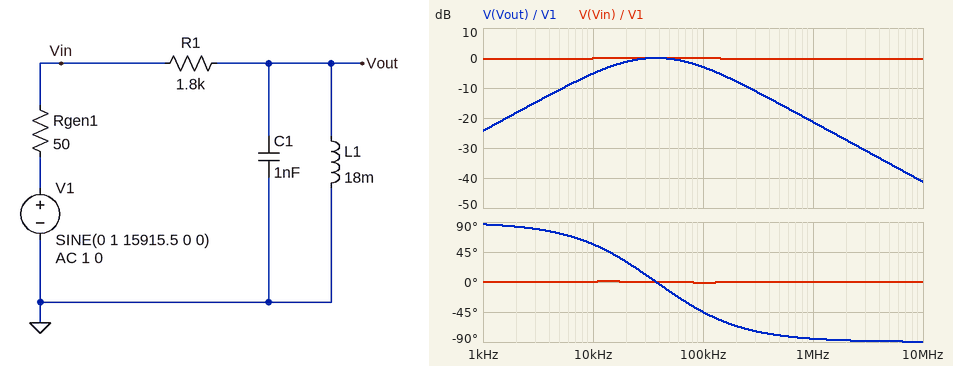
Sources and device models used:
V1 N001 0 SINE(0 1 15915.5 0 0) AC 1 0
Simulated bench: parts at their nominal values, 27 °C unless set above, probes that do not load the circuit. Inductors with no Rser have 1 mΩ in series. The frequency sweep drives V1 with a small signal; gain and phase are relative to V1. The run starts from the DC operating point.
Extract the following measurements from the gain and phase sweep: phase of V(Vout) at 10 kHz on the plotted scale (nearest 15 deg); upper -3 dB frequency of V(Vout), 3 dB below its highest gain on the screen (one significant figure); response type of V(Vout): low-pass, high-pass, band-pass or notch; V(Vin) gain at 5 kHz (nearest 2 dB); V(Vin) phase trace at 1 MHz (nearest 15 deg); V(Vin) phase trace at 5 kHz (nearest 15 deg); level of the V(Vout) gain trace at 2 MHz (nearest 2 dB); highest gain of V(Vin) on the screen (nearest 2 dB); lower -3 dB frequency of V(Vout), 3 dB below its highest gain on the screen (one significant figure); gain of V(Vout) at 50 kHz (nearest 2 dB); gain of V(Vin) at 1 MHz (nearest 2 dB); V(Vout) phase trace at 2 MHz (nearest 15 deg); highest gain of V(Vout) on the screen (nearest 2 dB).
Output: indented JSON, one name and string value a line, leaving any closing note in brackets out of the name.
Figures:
{
  "phase of V(Vout) at 10 kHz on the plotted scale": "60 deg",
  "upper -3 dB frequency of V(Vout), 3 dB below its highest gain on the screen": "100 kHz",
  "response type of V(Vout): low-pass, high-pass, band-pass or notch": "band-pass",
  "V(Vin) gain at 5 kHz": "0 dB",
  "V(Vin) phase trace at 1 MHz": "0 deg",
  "V(Vin) phase trace at 5 kHz": "0 deg",
  "level of the V(Vout) gain trace at 2 MHz": "-28 dB",
  "highest gain of V(Vin) on the screen": "0 dB",
  "lower -3 dB frequency of V(Vout), 3 dB below its highest gain on the screen": "10 kHz",
  "gain of V(Vout) at 50 kHz": "0 dB",
  "gain of V(Vin) at 1 MHz": "0 dB",
  "V(Vout) phase trace at 2 MHz": "-90 deg",
  "highest gain of V(Vout) on the screen": "0 dB"
}
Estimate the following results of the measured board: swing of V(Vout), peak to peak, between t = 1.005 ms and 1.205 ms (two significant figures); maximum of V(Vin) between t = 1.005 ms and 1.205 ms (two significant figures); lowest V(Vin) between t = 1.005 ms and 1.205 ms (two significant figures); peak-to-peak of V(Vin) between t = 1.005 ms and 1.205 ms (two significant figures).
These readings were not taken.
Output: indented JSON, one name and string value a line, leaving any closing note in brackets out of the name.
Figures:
{
  "swing of V(Vout), peak to peak, between t = 1.005 ms and 1.205 ms": "1.5 V",
  "maximum of V(Vin) between t = 1.005 ms and 1.205 ms": "990 mV",
  "lowest V(Vin) between t = 1.005 ms and 1.205 ms": "-990 mV",
  "peak-to-peak of V(Vin) between t = 1.005 ms and 1.205 ms": "2.0 V"
}
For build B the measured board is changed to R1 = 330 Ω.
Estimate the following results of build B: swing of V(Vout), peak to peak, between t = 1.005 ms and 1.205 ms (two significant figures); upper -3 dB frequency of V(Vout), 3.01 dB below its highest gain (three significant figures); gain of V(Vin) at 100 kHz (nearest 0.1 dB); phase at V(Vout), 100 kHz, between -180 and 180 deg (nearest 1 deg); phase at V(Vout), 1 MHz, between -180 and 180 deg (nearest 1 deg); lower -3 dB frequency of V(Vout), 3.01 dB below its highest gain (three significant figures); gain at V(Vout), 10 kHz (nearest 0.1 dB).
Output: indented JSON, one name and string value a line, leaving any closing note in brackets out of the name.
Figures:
{
  "swing of V(Vout), peak to peak, between t = 1.005 ms and 1.205 ms": "2.0 V",
  "upper -3 dB frequency of V(Vout), 3.01 dB below its highest gain": "422 kHz",
  "gain of V(Vin) at 100 kHz": "0 dB",
  "phase at V(Vout), 100 kHz, between -180 and 180 deg": "-12 deg",
  "phase at V(Vout), 1 MHz, between -180 and 180 deg": "-67 deg",
  "lower -3 dB frequency of V(Vout), 3.01 dB below its highest gain": "3.33 kHz",
  "gain at V(Vout), 10 kHz": "-0.4 dB"
}
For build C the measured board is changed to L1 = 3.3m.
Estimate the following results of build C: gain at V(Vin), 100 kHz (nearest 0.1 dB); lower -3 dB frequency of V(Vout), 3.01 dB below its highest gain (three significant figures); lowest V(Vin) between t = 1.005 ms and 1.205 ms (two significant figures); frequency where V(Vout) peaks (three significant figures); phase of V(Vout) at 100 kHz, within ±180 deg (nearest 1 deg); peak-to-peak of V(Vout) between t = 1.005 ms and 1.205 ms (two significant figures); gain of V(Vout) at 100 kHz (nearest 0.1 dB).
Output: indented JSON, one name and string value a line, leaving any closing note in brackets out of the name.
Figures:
{
  "gain at V(Vin), 100 kHz": "0 dB",
  "lower -3 dB frequency of V(Vout), 3.01 dB below its highest gain": "54.6 kHz",
  "lowest V(Vin) between t = 1.005 ms and 1.205 ms": "-970 mV",
  "frequency where V(Vout) peaks": "87.6 kHz",
  "phase of V(Vout) at 100 kHz, within ±180 deg": "-15 deg",
  "peak-to-peak of V(Vout) between t = 1.005 ms and 1.205 ms": "360 mV",
  "gain of V(Vout) at 100 kHz": "-0.3 dB"
}
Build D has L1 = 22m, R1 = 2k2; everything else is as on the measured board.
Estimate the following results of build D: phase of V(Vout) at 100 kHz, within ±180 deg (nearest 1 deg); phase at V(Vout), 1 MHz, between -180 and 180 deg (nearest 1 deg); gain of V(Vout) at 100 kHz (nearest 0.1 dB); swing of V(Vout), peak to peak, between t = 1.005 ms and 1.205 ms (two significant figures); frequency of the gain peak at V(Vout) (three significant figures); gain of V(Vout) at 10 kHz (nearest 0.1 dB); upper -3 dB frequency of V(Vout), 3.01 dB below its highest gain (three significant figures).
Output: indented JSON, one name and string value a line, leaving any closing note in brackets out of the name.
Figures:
{
  "phase of V(Vout) at 100 kHz, within ±180 deg": "-51 deg",
  "phase at V(Vout), 1 MHz, between -180 and 180 deg": "-86 deg",
  "gain of V(Vout) at 100 kHz": "-4.1 dB",
  "swing of V(Vout), peak to peak, between t = 1.005 ms and 1.205 ms": "1.6 V",
  "frequency of the gain peak at V(Vout)": "33.9 kHz",
  "gain of V(Vout) at 10 kHz": "-5.1 dB",
  "upper -3 dB frequency of V(Vout), 3.01 dB below its highest gain": "84.4 kHz"
}
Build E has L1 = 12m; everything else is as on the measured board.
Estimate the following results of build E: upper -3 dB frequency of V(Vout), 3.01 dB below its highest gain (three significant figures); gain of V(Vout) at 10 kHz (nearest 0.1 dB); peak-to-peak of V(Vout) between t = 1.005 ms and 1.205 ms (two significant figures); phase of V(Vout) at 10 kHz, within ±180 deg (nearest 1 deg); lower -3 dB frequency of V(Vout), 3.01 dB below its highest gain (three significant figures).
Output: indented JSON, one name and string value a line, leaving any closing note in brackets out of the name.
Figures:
{
  "upper -3 dB frequency of V(Vout), 3.01 dB below its highest gain": "106 kHz",
  "gain of V(Vout) at 10 kHz": "-8.1 dB",
  "peak-to-peak of V(Vout) between t = 1.005 ms and 1.205 ms": "1.2 V",
  "phase of V(Vout) at 10 kHz, within ±180 deg": "67 deg",
  "lower -3 dB frequency of V(Vout), 3.01 dB below its highest gain": "19.9 kHz"
}
